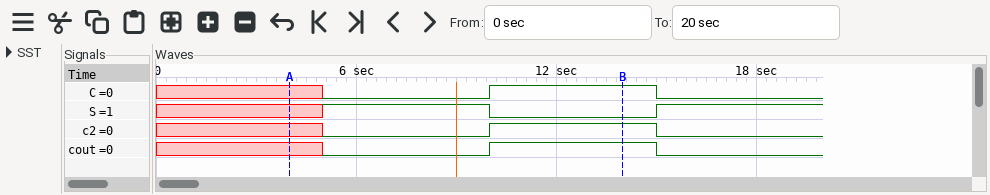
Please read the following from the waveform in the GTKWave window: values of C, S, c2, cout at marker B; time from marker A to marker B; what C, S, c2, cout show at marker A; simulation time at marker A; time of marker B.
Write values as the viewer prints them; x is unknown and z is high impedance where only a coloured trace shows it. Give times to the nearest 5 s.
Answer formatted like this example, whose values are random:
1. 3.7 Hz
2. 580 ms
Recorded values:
1. C=1, S=0, c2=1, cout=1
2. 10 s
3. C=x, S=x, c2=x, cout=x
4. 5 s
5. 15 s
